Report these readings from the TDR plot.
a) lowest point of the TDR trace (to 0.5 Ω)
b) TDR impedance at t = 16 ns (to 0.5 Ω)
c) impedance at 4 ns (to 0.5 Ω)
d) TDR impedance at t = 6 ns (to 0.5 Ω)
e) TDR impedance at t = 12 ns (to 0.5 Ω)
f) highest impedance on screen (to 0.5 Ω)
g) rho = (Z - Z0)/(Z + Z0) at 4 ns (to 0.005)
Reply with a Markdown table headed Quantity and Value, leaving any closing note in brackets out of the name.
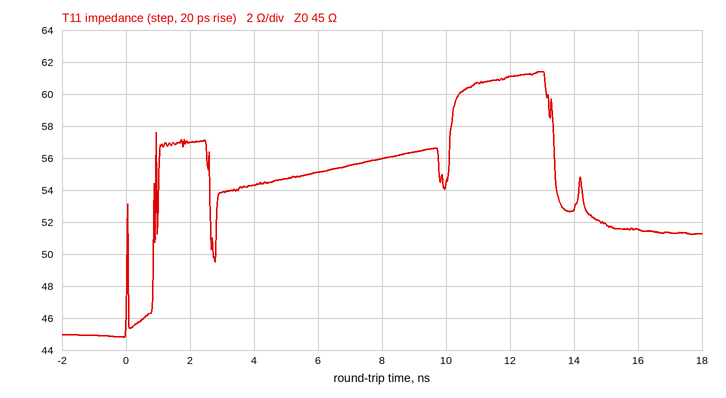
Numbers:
| Quantity | Value |
|---|---|
| lowest point of the TDR trace | 45.0 Ω |
| TDR impedance at t = 16 ns | 51.5 Ω |
| impedance at 4 ns | 54.5 Ω |
| TDR impedance at t = 6 ns | 55.0 Ω |
| TDR impedance at t = 12 ns | 61.0 Ω |
| highest impedance on screen | 61.5 Ω |
| rho = (Z - Z0)/(Z + Z0) at 4 ns | +0.095 |
